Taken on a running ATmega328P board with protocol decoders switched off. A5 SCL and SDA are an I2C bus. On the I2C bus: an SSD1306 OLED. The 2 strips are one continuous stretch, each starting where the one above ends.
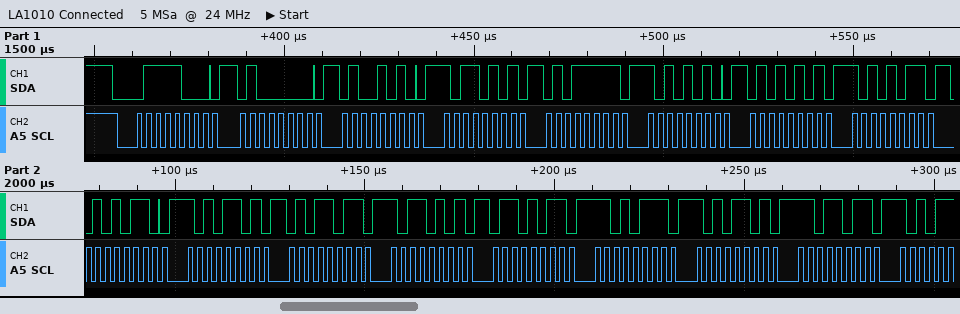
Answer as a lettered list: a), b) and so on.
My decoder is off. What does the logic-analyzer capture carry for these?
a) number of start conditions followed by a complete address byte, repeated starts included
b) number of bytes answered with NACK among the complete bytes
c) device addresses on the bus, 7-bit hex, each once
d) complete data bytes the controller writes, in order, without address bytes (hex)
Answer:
a) 1
b) 0
c) 0x3C
d) 40 4A B5 5F AA 55 AB 56 AD 5B B5 6B D7 AD DB
